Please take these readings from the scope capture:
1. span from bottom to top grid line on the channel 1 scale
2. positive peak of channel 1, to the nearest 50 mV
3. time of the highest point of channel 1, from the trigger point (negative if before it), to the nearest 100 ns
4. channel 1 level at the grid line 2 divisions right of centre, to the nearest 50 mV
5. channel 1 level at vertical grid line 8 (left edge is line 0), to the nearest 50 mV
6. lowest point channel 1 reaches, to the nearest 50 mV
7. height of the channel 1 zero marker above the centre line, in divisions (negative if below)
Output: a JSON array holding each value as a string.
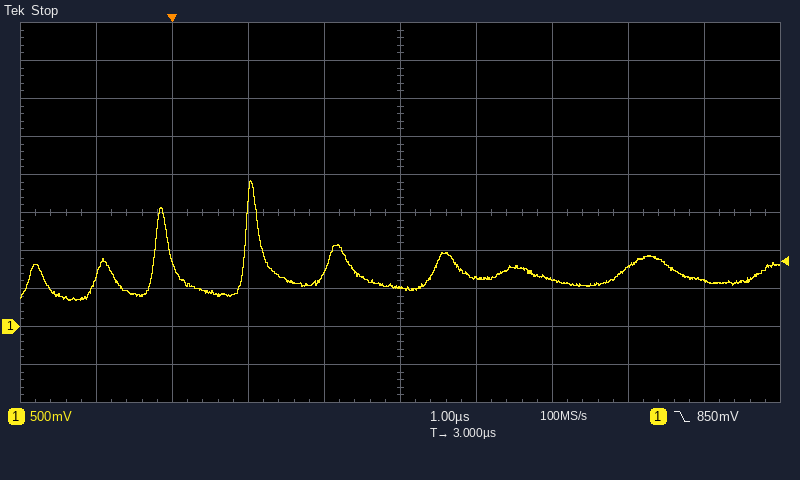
["5 V", "1.90 V", "+1.0 µs", "600 mV", "800 mV", "350 mV", "-3.0 div"]
